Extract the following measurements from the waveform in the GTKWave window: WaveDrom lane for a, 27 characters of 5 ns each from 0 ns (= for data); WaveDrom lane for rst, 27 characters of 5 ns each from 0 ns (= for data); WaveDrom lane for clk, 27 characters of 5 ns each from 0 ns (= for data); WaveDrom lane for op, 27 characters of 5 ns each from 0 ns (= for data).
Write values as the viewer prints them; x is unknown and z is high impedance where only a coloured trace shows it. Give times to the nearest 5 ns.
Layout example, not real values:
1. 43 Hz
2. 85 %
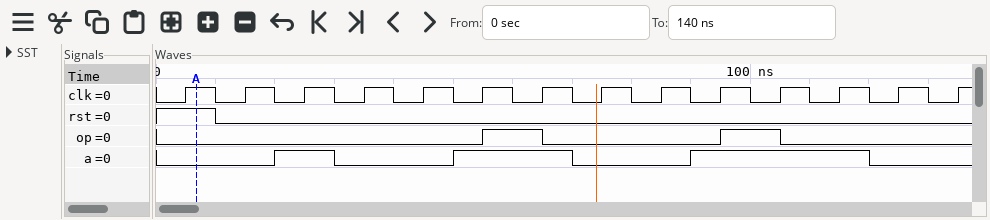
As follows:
1. {name: 'a', wave: '0...1.0...1...0...1.....0..'}
2. {name: 'rst', wave: '1.0........................'}
3. {name: 'clk', wave: '010101010101010101010101010'}
4. {name: 'op', wave: '0..........1.0.....1.0.....'}
